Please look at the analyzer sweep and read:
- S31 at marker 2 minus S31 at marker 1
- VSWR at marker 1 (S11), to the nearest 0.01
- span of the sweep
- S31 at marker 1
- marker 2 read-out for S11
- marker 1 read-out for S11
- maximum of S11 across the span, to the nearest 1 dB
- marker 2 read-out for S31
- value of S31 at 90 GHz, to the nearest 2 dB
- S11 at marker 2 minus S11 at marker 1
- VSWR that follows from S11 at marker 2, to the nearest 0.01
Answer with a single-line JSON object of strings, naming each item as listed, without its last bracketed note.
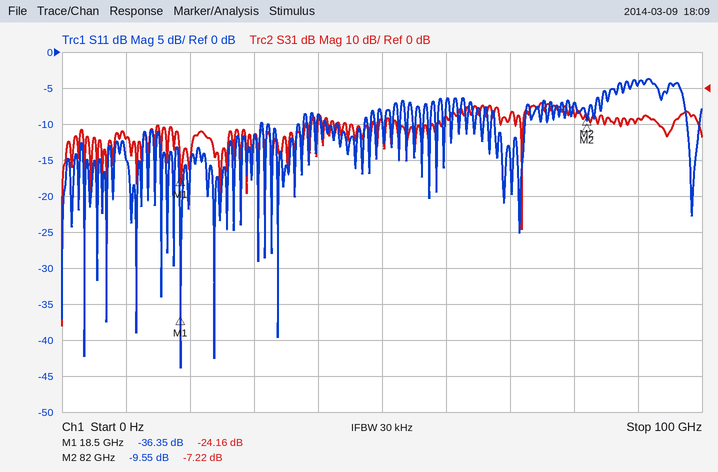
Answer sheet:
{"S31 at marker 2 minus S31 at marker 1": "16.94 dB", "VSWR at marker 1 (S11), to the nearest 0.01": "1.03", "span of the sweep": "100 GHz", "S31 at marker 1": "-24.16 dB", "marker 2 read-out for S11": "-9.55 dB", "marker 1 read-out for S11": "-36.35 dB", "maximum of S11 across the span, to the nearest 1 dB": "-4 dB", "marker 2 read-out for S31": "-7.22 dB", "value of S31 at 90 GHz, to the nearest 2 dB": "-8 dB", "S11 at marker 2 minus S11 at marker 1": "26.80 dB", "VSWR that follows from S11 at marker 2, to the nearest 0.01": "2.00"}
